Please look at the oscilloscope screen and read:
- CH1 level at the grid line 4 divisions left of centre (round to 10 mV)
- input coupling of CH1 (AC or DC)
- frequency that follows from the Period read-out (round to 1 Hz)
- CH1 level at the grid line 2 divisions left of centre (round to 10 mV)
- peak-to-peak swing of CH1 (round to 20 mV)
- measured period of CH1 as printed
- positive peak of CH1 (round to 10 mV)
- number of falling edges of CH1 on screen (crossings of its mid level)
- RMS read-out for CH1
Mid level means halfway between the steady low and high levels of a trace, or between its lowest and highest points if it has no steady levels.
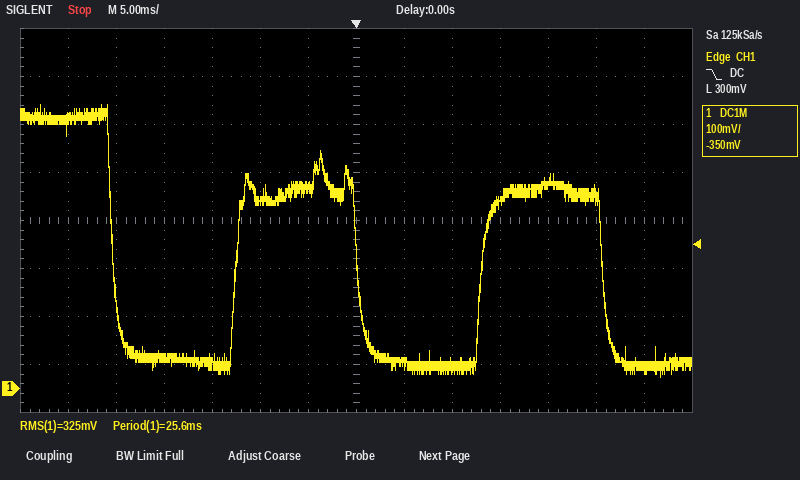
60 mV
DC
39 Hz
390 mV
560 mV
25.6 ms
590 mV
3
325 mV
